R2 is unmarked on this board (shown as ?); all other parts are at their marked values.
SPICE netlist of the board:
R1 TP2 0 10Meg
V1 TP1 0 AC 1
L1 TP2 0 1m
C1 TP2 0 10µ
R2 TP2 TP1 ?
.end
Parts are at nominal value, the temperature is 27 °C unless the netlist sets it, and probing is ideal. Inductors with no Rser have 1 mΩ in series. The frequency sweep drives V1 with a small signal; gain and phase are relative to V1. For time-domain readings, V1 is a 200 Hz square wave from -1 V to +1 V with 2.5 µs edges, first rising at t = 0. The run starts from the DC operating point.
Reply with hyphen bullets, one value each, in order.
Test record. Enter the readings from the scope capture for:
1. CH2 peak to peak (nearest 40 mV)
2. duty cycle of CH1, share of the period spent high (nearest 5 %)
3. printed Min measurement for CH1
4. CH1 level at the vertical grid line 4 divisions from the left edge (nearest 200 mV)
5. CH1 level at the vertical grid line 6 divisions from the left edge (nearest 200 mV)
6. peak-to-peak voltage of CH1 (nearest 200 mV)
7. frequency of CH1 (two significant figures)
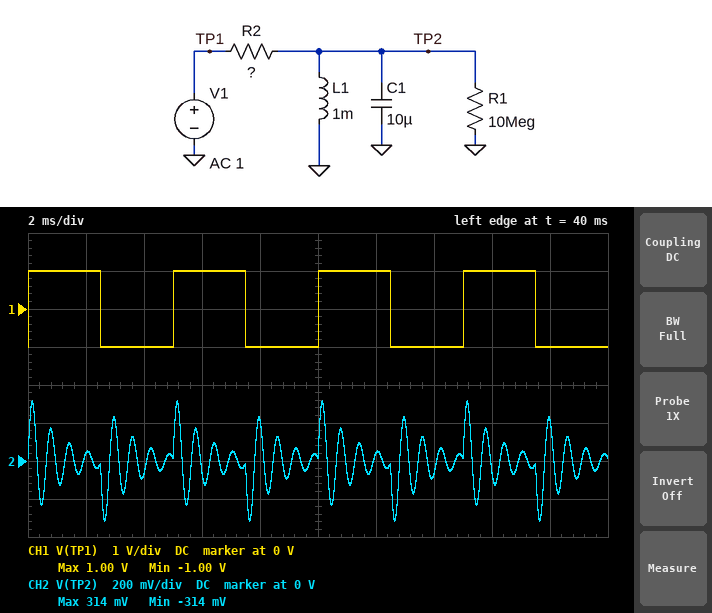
- 640 mV
- 50 %
- -1.00 V
- -1.0 V
- 1.0 V
- 2.0 V
- 200 Hz
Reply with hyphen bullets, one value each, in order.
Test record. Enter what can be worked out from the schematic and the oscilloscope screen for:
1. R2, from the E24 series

- 51 Ω
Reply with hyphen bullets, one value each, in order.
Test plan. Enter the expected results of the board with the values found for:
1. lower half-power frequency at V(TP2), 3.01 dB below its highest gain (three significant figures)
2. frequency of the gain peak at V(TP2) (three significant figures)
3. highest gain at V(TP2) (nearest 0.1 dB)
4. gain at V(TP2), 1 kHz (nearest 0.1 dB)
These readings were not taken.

- 1.44 kHz
- 1.59 kHz
- 0 dB
- -14.0 dB
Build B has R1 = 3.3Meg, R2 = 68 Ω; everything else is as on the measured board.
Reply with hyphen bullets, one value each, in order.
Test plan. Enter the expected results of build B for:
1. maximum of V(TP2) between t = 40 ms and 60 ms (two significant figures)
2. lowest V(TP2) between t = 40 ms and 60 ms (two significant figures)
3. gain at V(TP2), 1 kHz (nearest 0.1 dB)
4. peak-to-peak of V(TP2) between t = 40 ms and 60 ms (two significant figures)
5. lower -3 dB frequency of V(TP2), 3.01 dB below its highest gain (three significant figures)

- 230 mV
- -230 mV
- -16.4 dB
- 460 mV
- 1.48 kHz
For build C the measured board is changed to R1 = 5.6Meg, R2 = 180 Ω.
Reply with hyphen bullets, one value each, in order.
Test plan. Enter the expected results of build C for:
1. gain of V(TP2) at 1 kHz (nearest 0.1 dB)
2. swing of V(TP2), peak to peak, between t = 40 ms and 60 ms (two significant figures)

- -24.8 dB
- 140 mV
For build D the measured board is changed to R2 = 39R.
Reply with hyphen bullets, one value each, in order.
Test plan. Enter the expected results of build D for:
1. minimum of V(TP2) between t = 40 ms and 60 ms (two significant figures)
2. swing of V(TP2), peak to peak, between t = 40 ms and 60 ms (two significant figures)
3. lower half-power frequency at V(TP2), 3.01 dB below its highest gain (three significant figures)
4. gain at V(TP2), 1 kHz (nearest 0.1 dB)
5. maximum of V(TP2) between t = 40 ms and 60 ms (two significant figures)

- -410 mV
- 820 mV
- 1.40 kHz
- -11.8 dB
- 410 mV
